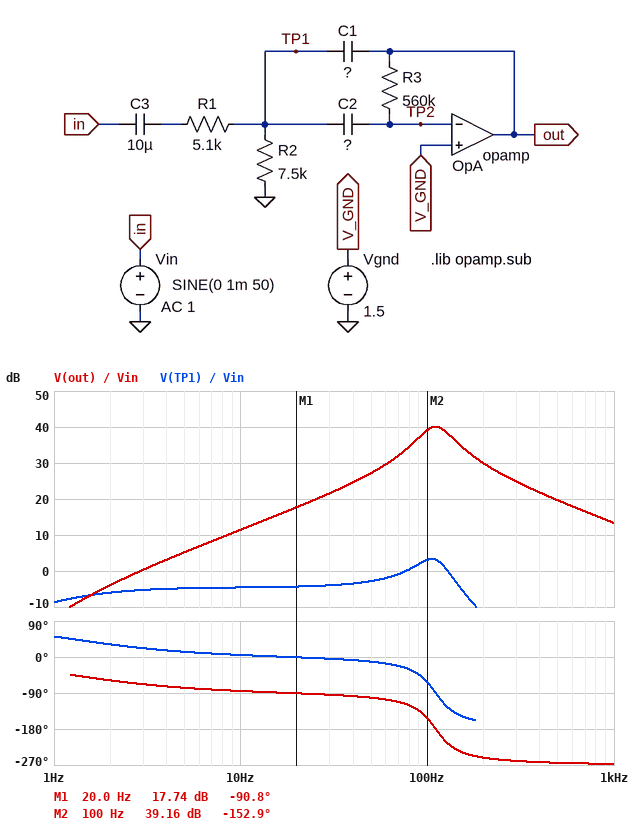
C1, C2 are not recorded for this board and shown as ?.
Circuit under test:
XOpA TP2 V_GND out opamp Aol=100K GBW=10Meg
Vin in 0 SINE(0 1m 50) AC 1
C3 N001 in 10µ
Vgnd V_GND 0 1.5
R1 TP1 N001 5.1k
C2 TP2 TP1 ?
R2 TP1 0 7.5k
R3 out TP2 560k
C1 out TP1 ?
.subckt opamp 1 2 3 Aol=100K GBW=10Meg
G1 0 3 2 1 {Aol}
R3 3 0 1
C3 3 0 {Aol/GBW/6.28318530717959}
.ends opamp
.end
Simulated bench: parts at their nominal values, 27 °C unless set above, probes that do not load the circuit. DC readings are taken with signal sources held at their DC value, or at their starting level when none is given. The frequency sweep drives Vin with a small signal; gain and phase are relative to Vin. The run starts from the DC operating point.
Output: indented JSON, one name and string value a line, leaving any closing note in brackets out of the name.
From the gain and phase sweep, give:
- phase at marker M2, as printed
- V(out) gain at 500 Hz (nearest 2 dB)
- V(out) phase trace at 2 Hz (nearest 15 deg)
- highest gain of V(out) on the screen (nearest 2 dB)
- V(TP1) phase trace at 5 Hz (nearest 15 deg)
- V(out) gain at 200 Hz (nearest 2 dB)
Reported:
{
  "phase at marker M2, as printed": "-152.9 deg",
  "V(out) gain at 500 Hz": "20 dB",
  "V(out) phase trace at 2 Hz": "-60 deg",
  "highest gain of V(out) on the screen": "40 dB",
  "V(TP1) phase trace at 5 Hz": "15 deg",
  "V(out) gain at 200 Hz": "30 dB"
}
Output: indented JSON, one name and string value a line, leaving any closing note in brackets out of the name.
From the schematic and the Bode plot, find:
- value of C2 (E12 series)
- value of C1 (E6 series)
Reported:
{
  "value of C2": "180 nF",
  "value of C1": "6.8 nF"
}
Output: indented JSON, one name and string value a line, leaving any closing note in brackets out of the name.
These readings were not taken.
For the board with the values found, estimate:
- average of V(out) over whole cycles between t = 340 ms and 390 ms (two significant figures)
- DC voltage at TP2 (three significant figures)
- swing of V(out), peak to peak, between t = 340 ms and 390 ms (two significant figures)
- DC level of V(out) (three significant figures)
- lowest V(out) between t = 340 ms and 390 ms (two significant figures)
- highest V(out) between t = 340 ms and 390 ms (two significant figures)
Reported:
{
  "average of V(out) over whole cycles between t = 340 ms and 390 ms": "1.5 V",
  "DC voltage at TP2": "1.50 V",
  "swing of V(out), peak to peak, between t = 340 ms and 390 ms": "46 mV",
  "DC level of V(out)": "1.50 V",
  "lowest V(out) between t = 340 ms and 390 ms": "1.5 V",
  "highest V(out) between t = 340 ms and 390 ms": "1.5 V"
}
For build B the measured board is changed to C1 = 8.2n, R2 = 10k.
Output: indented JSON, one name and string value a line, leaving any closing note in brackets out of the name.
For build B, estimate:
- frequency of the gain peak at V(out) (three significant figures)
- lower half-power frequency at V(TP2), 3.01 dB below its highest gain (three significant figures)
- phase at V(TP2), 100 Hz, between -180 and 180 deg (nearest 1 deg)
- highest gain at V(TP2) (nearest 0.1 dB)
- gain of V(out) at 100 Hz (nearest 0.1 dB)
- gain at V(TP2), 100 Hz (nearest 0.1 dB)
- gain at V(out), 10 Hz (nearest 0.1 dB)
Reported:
{
  "frequency of the gain peak at V(out)": "95.6 Hz",
  "lower half-power frequency at V(TP2), 3.01 dB below its highest gain": "80.8 Hz",
  "phase at V(TP2), 100 Hz, between -180 and 180 deg": "33 deg",
  "highest gain at V(TP2)": "-57.2 dB",
  "gain of V(out) at 100 Hz": "39.7 dB",
  "gain at V(TP2), 100 Hz": "-57.3 dB",
  "gain at V(out), 10 Hz": "12.4 dB"
}
